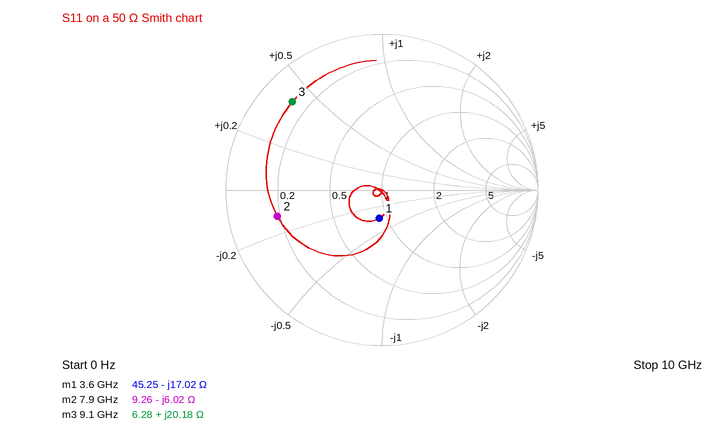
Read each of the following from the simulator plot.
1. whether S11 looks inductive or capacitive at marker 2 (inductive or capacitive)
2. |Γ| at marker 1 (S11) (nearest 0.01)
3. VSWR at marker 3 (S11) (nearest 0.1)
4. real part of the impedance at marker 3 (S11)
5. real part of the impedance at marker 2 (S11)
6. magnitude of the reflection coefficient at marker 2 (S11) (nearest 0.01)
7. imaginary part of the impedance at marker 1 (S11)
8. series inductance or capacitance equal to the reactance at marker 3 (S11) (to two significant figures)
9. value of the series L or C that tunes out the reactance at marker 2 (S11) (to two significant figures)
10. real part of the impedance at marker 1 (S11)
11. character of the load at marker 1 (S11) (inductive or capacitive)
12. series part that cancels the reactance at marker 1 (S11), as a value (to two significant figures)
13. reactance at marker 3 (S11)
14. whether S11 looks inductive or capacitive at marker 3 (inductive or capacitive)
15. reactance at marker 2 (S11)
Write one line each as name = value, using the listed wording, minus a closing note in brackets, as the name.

whether S11 looks inductive or capacitive at marker 2 = capacitive
|Γ| at marker 1 (S11) = 0.18
VSWR at marker 3 (S11) = 9.3
real part of the impedance at marker 3 = 6.28 Ω
real part of the impedance at marker 2 = 9.26 Ω
magnitude of the reflection coefficient at marker 2 (S11) = 0.69
imaginary part of the impedance at marker 1 = -17.02 Ω
series inductance or capacitance equal to the reactance at marker 3 (S11) = 350 pH
value of the series L or C that tunes out the reactance at marker 2 (S11) = 120 pH
real part of the impedance at marker 1 = 45.25 Ω
character of the load at marker 1 (S11) = capacitive
series part that cancels the reactance at marker 1 (S11), as a value = 750 pH
reactance at marker 3 = +20.18 Ω
whether S11 looks inductive or capacitive at marker 3 = inductive
reactance at marker 2 = -6.02 Ω
